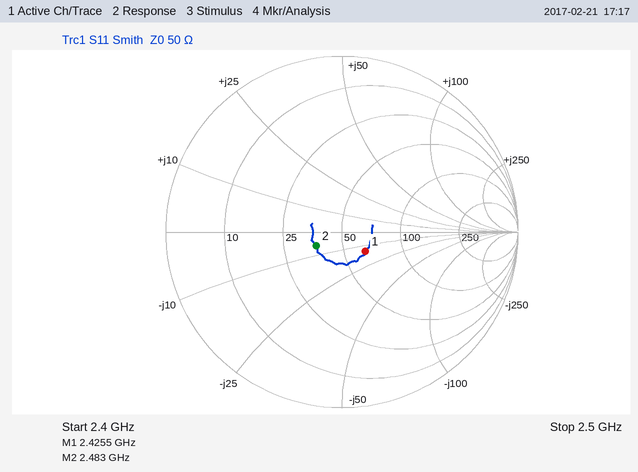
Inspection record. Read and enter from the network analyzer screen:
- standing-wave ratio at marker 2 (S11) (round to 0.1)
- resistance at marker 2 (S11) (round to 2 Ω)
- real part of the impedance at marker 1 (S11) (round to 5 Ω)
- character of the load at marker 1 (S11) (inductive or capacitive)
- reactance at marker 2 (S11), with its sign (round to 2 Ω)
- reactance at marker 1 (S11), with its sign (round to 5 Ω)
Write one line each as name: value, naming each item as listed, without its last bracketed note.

standing-wave ratio at marker 2 (S11): 1.4
resistance at marker 2 (S11): 36 Ω
real part of the impedance at marker 1 (S11): 65 Ω
character of the load at marker 1 (S11): capacitive
reactance at marker 2 (S11), with its sign: -6 Ω
reactance at marker 1 (S11), with its sign: -15 Ω
